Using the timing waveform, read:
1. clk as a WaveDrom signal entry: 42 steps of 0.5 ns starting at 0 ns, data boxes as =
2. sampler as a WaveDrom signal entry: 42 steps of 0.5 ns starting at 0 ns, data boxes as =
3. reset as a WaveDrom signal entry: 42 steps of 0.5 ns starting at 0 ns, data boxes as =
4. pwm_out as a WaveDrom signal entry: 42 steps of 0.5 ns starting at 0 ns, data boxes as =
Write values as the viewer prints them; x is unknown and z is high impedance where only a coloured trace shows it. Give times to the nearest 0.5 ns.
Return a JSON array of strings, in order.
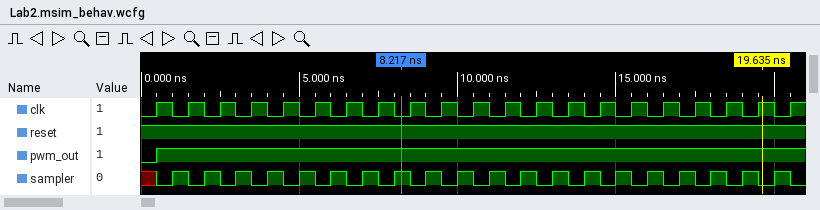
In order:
["{name: 'clk', wave: '010101010101010101010101010101010101010101'}", "{name: 'sampler', wave: 'x01010101010101010101010101010101010101010'}", "{name: 'reset', wave: '1.........................................'}", "{name: 'pwm_out', wave: '01........................................'}"]
